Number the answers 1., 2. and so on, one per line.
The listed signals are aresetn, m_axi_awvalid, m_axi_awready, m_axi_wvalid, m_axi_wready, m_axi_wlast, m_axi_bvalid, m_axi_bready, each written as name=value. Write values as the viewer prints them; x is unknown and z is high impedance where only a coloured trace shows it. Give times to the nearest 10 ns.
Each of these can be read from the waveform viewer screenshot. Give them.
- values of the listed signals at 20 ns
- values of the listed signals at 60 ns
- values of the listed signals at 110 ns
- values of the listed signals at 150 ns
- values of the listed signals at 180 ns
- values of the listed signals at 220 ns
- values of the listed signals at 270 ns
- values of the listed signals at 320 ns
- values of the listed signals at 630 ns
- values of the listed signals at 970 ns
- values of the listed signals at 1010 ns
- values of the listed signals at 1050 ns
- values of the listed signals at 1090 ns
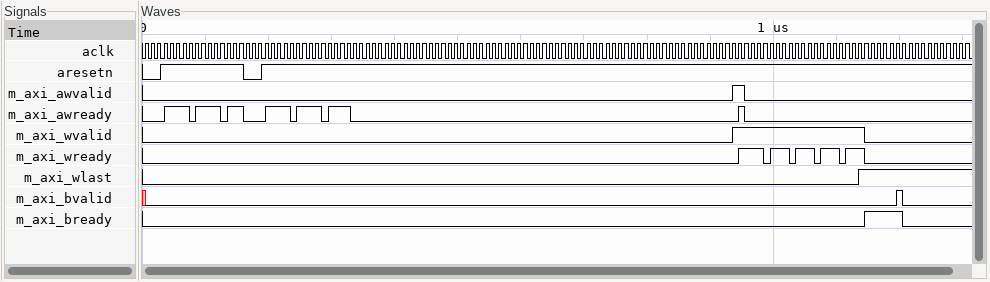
1. aresetn=0, m_axi_awvalid=0, m_axi_awready=0, m_axi_wvalid=0, m_axi_wready=0, m_axi_wlast=0, m_axi_bvalid=0, m_axi_bready=0
2. aresetn=1, m_axi_awvalid=0, m_axi_awready=1, m_axi_wvalid=0, m_axi_wready=0, m_axi_wlast=0, m_axi_bvalid=0, m_axi_bready=0
3. aresetn=1, m_axi_awvalid=0, m_axi_awready=1, m_axi_wvalid=0, m_axi_wready=0, m_axi_wlast=0, m_axi_bvalid=0, m_axi_bready=0
4. aresetn=1, m_axi_awvalid=0, m_axi_awready=1, m_axi_wvalid=0, m_axi_wready=0, m_axi_wlast=0, m_axi_bvalid=0, m_axi_bready=0
5. aresetn=0, m_axi_awvalid=0, m_axi_awready=0, m_axi_wvalid=0, m_axi_wready=0, m_axi_wlast=0, m_axi_bvalid=0, m_axi_bready=0
6. aresetn=1, m_axi_awvalid=0, m_axi_awready=1, m_axi_wvalid=0, m_axi_wready=0, m_axi_wlast=0, m_axi_bvalid=0, m_axi_bready=0
7. aresetn=1, m_axi_awvalid=0, m_axi_awready=1, m_axi_wvalid=0, m_axi_wready=0, m_axi_wlast=0, m_axi_bvalid=0, m_axi_bready=0
8. aresetn=1, m_axi_awvalid=0, m_axi_awready=1, m_axi_wvalid=0, m_axi_wready=0, m_axi_wlast=0, m_axi_bvalid=0, m_axi_bready=0
9. aresetn=1, m_axi_awvalid=0, m_axi_awready=0, m_axi_wvalid=0, m_axi_wready=0, m_axi_wlast=0, m_axi_bvalid=0, m_axi_bready=0
10. aresetn=1, m_axi_awvalid=0, m_axi_awready=0, m_axi_wvalid=1, m_axi_wready=1, m_axi_wlast=0, m_axi_bvalid=0, m_axi_bready=0
11. aresetn=1, m_axi_awvalid=0, m_axi_awready=0, m_axi_wvalid=1, m_axi_wready=1, m_axi_wlast=0, m_axi_bvalid=0, m_axi_bready=0
12. aresetn=1, m_axi_awvalid=0, m_axi_awready=0, m_axi_wvalid=1, m_axi_wready=1, m_axi_wlast=0, m_axi_bvalid=0, m_axi_bready=0
13. aresetn=1, m_axi_awvalid=0, m_axi_awready=0, m_axi_wvalid=1, m_axi_wready=1, m_axi_wlast=0, m_axi_bvalid=0, m_axi_bready=0
